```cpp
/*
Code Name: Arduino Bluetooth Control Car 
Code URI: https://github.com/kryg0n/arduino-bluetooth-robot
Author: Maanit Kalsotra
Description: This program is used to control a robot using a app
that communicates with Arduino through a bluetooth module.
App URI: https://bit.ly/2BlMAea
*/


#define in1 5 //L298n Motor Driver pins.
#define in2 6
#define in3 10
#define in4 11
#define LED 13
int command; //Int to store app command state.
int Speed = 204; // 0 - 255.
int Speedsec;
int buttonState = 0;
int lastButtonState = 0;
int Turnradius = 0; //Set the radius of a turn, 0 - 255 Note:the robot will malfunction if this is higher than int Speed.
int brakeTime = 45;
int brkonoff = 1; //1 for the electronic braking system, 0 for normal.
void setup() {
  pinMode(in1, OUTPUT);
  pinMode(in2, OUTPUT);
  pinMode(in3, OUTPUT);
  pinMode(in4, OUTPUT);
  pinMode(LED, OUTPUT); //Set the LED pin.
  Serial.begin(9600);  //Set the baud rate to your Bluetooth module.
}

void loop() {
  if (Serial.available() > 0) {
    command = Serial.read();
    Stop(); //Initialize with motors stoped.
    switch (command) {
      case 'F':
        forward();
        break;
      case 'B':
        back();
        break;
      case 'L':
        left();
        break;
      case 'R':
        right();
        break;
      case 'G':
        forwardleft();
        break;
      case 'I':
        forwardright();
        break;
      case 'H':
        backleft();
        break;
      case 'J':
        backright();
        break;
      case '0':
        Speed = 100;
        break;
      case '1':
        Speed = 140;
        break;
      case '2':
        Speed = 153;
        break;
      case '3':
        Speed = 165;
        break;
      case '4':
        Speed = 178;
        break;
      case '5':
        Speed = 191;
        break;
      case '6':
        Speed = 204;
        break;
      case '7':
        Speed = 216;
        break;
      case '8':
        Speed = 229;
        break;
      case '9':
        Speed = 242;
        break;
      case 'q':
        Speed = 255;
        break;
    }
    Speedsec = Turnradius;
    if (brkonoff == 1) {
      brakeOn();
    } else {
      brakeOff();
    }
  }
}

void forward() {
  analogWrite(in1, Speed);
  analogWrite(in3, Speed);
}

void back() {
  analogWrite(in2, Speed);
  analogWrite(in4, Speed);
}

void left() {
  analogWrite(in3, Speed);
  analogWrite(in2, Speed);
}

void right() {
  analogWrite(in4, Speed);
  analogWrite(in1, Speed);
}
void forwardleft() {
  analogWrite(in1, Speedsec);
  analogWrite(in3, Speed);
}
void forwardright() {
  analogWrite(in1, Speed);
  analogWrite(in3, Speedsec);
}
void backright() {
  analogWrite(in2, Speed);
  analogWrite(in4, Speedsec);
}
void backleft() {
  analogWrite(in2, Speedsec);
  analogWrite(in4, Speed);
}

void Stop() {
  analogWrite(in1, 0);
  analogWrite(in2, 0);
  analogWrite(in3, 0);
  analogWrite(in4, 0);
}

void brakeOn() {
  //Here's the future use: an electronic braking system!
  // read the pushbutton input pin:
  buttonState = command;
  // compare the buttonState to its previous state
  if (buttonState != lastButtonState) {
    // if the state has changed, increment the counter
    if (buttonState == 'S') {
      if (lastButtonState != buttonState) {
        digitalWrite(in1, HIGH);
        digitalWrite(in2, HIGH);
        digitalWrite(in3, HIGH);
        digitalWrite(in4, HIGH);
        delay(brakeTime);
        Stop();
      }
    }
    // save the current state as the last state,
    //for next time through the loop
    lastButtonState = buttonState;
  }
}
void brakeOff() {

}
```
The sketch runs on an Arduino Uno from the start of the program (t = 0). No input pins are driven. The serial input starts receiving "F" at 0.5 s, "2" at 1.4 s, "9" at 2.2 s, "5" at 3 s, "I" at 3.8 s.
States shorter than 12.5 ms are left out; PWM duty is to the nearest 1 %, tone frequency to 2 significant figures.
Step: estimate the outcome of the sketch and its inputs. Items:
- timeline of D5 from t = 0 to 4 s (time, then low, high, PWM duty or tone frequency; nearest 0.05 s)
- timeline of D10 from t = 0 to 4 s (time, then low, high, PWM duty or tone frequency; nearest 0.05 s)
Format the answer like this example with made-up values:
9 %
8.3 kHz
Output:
0 s low; 0.5 s PWM 80 %; 1.4 s low; 3.8 s PWM 75 %
0 s low; 0.5 s PWM 80 %; 1.4 s low
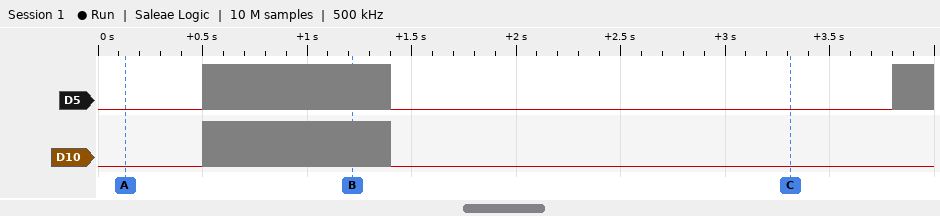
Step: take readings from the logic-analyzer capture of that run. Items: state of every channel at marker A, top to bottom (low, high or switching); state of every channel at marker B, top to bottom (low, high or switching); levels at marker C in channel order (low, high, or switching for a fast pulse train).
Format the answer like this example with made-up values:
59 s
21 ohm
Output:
D5 low, D10 low
D5 switching, D10 switching
D5 low, D10 low
